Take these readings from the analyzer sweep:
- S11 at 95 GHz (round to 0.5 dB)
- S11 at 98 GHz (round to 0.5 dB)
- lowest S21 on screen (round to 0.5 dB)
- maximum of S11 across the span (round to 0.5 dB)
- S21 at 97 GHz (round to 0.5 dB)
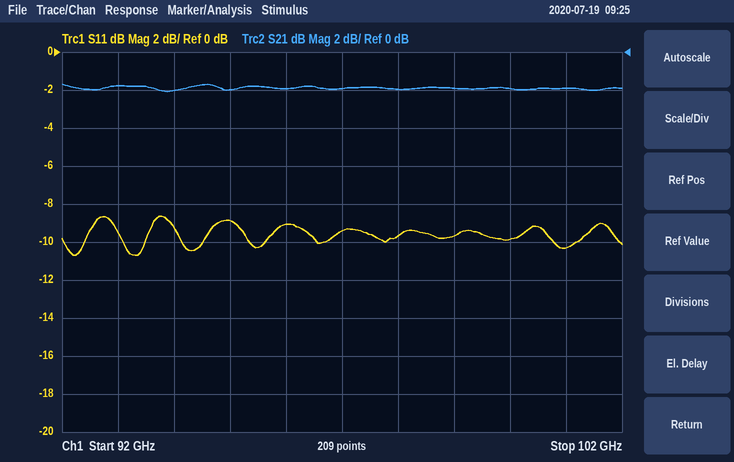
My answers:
-9.0 dB
-9.5 dB
-2.0 dB
-8.5 dB
-2.0 dB
